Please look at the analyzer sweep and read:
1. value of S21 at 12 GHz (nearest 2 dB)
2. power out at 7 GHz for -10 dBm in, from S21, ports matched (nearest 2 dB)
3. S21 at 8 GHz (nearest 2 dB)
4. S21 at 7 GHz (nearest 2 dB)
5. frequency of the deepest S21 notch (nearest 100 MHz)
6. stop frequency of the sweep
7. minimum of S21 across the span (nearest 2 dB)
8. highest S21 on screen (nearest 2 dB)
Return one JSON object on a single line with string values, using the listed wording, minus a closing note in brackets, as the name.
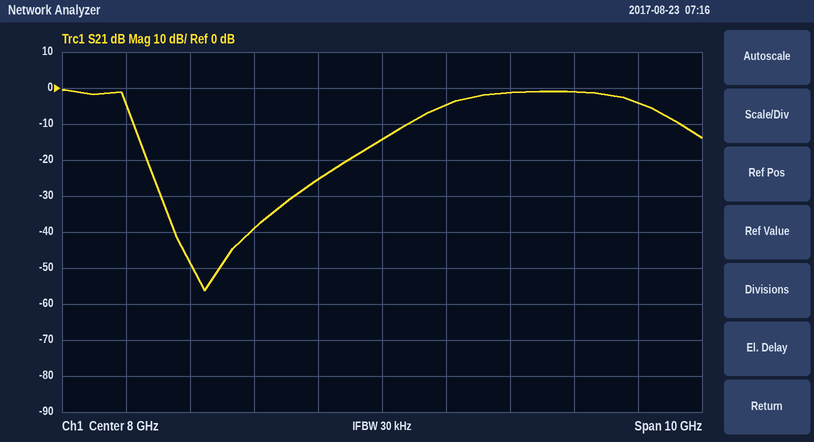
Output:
{"value of S21 at 12 GHz": "-4 dB", "power out at 7 GHz for -10 dBm in, from S21, ports matched": "-36 dBm", "S21 at 8 GHz": "-14 dB", "S21 at 7 GHz": "-26 dB", "frequency of the deepest S21 notch": "5.2 GHz", "stop frequency of the sweep": "13 GHz", "minimum of S21 across the span": "-56 dB", "highest S21 on screen": "0 dB"}
